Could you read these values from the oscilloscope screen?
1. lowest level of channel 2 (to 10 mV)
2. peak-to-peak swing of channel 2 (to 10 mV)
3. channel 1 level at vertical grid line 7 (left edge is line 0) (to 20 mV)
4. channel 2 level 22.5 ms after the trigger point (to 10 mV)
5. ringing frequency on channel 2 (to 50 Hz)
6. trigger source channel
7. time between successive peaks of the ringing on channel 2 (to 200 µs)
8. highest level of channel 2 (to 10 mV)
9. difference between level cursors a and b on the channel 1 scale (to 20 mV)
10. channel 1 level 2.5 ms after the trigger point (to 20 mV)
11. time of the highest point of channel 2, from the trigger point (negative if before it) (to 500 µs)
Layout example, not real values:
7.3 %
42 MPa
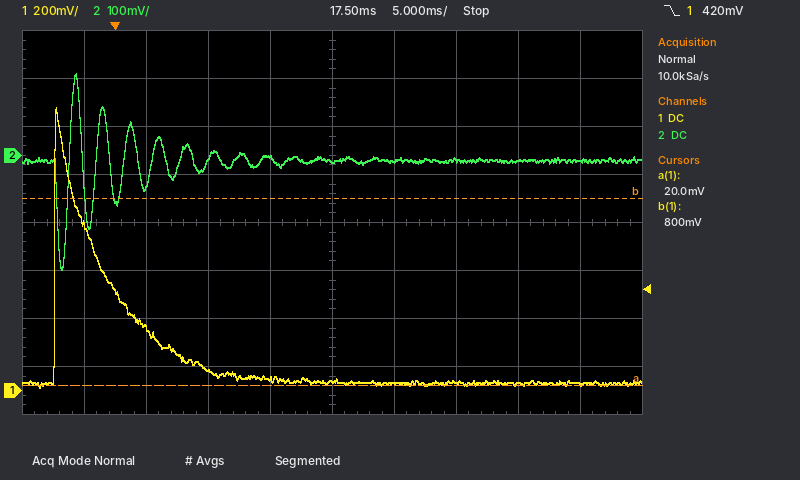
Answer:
-240 mV
410 mV
40 mV
-10 mV
450 Hz
channel 1
2.2 ms
170 mV
780 mV
260 mV
-3.0 ms
